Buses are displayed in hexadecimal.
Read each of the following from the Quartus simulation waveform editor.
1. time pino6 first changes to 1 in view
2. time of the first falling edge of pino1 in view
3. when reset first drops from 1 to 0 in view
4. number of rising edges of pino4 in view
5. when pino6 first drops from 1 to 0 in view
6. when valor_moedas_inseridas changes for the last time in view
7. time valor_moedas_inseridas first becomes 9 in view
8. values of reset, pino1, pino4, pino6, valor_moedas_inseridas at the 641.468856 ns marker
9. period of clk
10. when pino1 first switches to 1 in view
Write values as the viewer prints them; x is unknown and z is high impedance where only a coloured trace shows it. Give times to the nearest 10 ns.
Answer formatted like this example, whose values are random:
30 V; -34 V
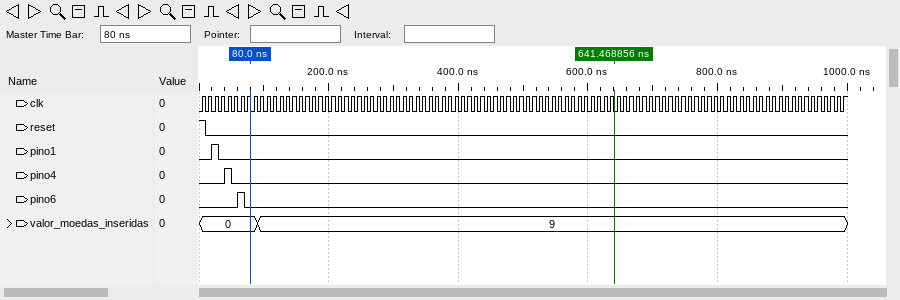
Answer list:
60 ns; 30 ns; 10 ns; 1; 70 ns; 90 ns; 90 ns; reset=0, pino1=0, pino4=0, pino6=0, valor_moedas_inseridas=9; 10 ns; 20 ns
